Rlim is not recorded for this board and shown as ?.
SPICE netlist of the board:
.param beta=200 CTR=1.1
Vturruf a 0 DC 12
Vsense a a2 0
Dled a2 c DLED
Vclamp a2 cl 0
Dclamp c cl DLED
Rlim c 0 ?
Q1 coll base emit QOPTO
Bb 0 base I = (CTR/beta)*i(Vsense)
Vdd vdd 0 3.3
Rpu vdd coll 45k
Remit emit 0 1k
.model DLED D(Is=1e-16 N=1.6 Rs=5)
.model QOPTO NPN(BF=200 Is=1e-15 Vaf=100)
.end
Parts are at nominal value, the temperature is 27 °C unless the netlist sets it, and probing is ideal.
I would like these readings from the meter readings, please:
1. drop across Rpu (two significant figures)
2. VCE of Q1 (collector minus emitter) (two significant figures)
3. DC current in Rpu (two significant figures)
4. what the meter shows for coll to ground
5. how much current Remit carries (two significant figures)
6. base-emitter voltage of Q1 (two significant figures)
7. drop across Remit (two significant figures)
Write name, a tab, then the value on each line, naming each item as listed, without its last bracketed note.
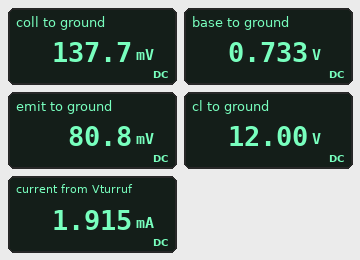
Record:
drop across Rpu	3.2 V
VCE of Q1 (collector minus emitter)	57 mV
DC current in Rpu	70 µA
what the meter shows for coll to ground	137.7 mV
how much current Remit carries	81 µA
base-emitter voltage of Q1	650 mV
drop across Remit	81 mV
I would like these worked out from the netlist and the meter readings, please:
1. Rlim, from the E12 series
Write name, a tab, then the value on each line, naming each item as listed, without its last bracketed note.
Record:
Rlim, from the E12 series	5.6 kΩ
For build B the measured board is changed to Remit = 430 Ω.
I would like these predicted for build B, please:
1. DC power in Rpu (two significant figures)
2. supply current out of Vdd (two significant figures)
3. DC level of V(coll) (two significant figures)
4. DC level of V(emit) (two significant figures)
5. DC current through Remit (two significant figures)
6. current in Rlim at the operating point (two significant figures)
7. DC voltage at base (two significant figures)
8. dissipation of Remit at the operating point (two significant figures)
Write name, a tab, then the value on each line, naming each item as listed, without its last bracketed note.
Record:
DC power in Rpu	230 µW
supply current out of Vdd	71 µA
DC level of V(coll)	92 mV
DC level of V(emit)	35 mV
DC current through Remit	82 µA
current in Rlim at the operating point	1.9 mA
DC voltage at base	690 mV
dissipation of Remit at the operating point	2.9 µW
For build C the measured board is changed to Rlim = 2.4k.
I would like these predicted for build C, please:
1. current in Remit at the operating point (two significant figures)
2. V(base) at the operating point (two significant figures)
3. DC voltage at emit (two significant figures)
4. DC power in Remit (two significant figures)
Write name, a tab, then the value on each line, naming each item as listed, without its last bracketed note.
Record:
current in Remit at the operating point	95 µA
V(base) at the operating point	750 mV
DC voltage at emit	95 mV
DC power in Remit	9.0 µW
